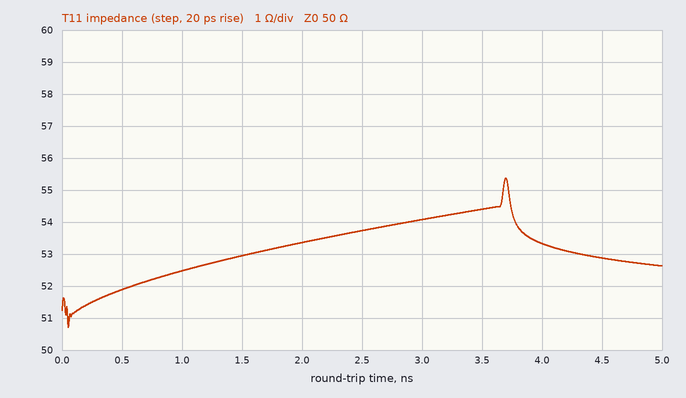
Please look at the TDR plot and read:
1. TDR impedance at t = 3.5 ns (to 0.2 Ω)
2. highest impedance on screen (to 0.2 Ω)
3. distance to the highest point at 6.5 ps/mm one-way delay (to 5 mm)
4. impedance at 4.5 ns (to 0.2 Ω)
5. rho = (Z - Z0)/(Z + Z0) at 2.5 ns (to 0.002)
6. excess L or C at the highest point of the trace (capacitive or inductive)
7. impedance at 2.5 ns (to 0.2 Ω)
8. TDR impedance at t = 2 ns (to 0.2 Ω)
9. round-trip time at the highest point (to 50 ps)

54.4 Ω
55.4 Ω
285 mm
52.8 Ω
+0.036
inductive
53.8 Ω
53.4 Ω
3.70 ns
